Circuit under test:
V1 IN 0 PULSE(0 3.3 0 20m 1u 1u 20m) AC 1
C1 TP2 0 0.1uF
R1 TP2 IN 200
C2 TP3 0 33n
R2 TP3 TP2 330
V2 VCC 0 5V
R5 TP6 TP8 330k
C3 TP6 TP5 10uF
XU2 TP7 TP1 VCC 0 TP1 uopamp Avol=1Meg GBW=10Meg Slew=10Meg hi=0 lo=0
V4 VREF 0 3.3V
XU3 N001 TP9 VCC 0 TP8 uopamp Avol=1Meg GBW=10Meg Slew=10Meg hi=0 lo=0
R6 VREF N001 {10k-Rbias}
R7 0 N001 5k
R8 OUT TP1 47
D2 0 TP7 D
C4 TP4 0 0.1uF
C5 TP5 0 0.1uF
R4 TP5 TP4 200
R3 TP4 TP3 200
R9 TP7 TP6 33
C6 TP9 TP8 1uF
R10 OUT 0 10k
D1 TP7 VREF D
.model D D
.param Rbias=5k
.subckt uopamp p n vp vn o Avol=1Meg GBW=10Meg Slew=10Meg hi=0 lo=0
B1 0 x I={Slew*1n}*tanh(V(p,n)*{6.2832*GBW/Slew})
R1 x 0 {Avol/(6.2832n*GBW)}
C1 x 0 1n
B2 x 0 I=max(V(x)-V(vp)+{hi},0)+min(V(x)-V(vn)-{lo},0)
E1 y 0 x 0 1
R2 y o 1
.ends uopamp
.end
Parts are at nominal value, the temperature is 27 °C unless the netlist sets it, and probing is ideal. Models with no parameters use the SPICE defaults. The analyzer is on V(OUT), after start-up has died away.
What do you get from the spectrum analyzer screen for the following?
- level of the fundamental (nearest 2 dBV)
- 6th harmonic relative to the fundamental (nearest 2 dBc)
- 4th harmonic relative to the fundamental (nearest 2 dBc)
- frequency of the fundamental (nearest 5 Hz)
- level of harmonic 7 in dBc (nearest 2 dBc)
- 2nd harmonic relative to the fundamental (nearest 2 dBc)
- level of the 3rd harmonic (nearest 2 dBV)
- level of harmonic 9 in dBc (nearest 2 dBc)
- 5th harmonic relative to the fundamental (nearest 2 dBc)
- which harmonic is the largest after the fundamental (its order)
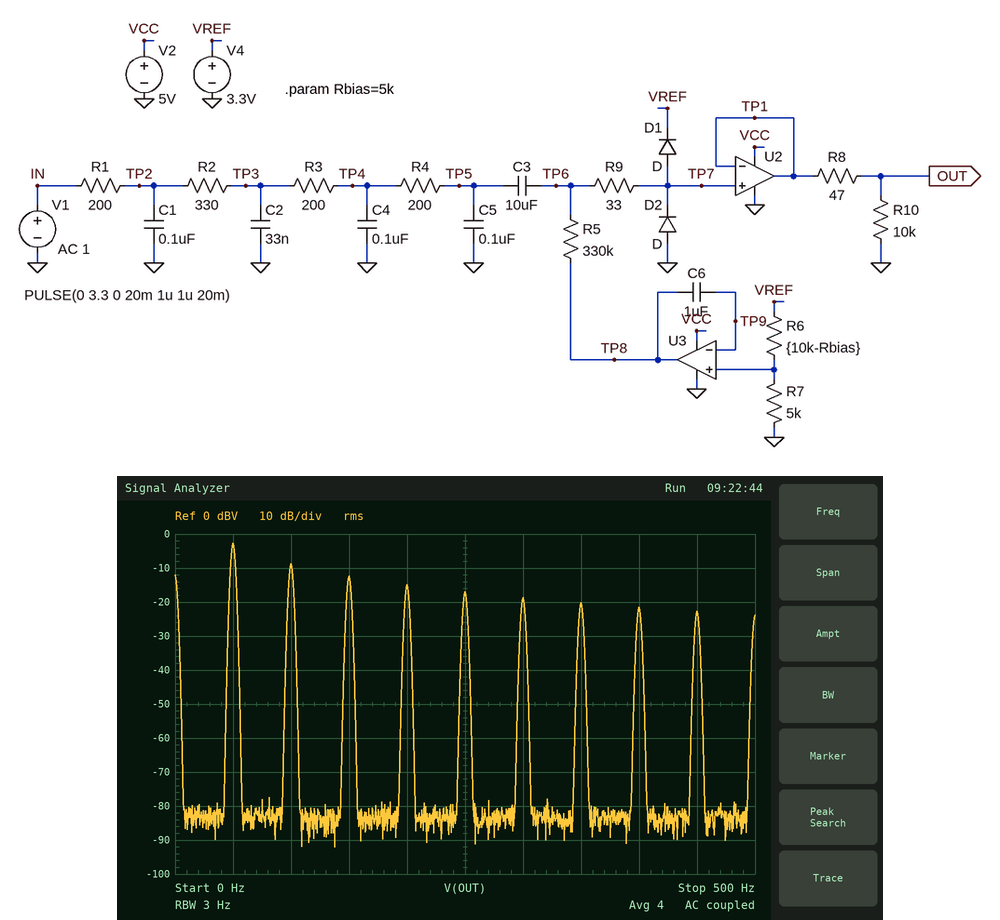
-2 dBV
-16 dBc
-12 dBc
50 Hz
-18 dBc
-6 dBc
-12 dBV
-20 dBc
-14 dBc
2
